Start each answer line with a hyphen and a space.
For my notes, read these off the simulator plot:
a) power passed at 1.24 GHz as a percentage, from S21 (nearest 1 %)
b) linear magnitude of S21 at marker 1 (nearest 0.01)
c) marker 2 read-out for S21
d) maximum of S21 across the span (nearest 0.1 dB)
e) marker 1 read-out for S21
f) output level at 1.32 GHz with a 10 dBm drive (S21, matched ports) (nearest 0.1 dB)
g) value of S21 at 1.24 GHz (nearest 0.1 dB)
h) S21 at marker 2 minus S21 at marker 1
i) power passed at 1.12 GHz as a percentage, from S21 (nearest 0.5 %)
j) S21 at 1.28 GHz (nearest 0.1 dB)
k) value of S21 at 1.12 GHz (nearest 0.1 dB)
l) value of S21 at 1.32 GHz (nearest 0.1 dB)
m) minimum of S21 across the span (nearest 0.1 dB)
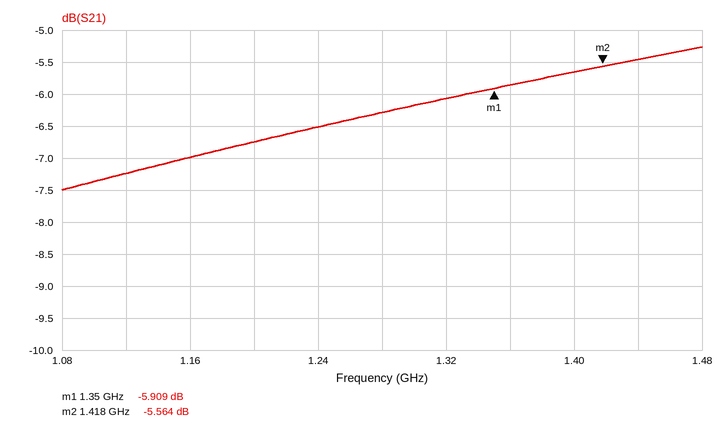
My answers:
- 22 %
- 0.51
- -5.564 dB
- -5.3 dB
- -5.909 dB
- 3.9 dBm
- -6.5 dB
- 0.345 dB
- 19.0 %
- -6.3 dB
- -7.2 dB
- -6.1 dB
- -7.5 dB
